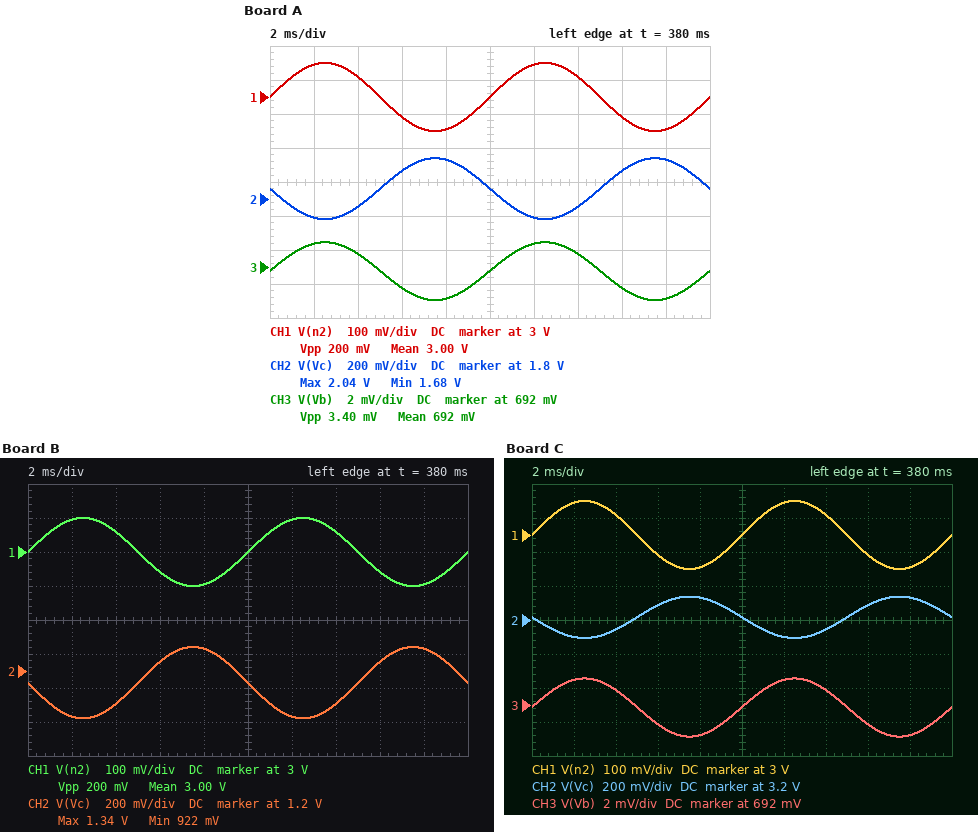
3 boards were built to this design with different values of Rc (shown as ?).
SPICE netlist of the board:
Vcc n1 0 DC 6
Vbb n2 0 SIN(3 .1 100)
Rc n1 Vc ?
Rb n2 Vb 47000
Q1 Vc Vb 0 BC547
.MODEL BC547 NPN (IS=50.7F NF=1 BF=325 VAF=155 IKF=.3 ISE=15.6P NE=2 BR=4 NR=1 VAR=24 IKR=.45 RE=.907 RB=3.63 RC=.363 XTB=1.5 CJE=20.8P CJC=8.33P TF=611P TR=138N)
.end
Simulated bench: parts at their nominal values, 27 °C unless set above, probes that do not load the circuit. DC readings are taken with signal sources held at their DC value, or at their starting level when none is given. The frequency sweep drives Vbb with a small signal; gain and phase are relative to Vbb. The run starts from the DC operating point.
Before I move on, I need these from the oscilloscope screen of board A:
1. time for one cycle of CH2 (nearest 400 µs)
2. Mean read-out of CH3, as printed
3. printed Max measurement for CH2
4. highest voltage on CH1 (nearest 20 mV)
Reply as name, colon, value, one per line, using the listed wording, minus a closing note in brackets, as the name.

time for one cycle of CH2: 10.0 ms
Mean read-out of CH3, as printed: 692 mV
printed Max measurement for CH2: 2.04 V
highest voltage on CH1: 3.10 V
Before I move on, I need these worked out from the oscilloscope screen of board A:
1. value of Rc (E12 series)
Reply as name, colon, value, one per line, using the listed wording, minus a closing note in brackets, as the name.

value of Rc: 330 Ω
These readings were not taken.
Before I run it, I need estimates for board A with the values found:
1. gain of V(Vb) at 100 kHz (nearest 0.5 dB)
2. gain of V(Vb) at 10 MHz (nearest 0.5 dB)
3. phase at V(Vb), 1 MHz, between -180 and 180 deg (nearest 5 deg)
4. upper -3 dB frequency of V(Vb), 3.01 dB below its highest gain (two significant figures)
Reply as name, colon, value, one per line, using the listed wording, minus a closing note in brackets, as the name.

gain of V(Vb) at 100 kHz: -36.0 dB
gain of V(Vb) at 10 MHz: -68.0 dB
phase at V(Vb), 1 MHz, between -180 and 180 deg: -75 deg
upper -3 dB frequency of V(Vb), 3.01 dB below its highest gain: 230 kHz
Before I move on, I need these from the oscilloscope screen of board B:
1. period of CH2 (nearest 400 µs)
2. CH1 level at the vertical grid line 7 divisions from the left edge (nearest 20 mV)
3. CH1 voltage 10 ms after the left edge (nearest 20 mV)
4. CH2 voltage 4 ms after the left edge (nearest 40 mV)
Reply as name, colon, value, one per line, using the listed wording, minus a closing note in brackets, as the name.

period of CH2: 10.0 ms
CH1 level at the vertical grid line 7 divisions from the left edge: 3.06 V
CH1 voltage 10 ms after the left edge: 3.00 V
CH2 voltage 4 ms after the left edge: 1.00 V
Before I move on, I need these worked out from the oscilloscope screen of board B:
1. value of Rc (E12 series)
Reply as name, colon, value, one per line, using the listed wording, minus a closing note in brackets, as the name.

value of Rc: 390 Ω
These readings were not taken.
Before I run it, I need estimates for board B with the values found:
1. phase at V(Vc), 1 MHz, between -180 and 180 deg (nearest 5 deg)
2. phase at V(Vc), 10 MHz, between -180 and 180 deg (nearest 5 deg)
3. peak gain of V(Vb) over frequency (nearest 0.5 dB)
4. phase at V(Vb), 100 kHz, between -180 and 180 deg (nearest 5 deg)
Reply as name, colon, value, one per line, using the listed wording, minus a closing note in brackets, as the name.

phase at V(Vc), 1 MHz, between -180 and 180 deg: 100 deg
phase at V(Vc), 10 MHz, between -180 and 180 deg: 90 deg
peak gain of V(Vb) over frequency: -35.5 dB
phase at V(Vb), 100 kHz, between -180 and 180 deg: -30 deg
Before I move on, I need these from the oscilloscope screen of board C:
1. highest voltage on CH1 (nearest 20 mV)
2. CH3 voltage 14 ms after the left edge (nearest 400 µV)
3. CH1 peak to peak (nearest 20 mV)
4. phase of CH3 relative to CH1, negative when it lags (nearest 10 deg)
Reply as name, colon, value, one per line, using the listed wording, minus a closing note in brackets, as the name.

highest voltage on CH1: 3.10 V
CH3 voltage 14 ms after the left edge: 692.8 mV
CH1 peak to peak: 200 mV
phase of CH3 relative to CH1, negative when it lags: 0 deg
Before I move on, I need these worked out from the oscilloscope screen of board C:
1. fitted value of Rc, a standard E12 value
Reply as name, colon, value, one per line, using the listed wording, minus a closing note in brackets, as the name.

fitted value of Rc, a standard E12 value: 220 Ω
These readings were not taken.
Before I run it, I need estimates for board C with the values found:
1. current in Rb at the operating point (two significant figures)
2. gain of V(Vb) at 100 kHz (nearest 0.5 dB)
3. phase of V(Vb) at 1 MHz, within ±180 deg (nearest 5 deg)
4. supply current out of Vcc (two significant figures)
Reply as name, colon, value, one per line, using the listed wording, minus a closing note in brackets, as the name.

current in Rb at the operating point: 49 µA
gain of V(Vb) at 100 kHz: -35.5 dB
phase of V(Vb) at 1 MHz, within ±180 deg: -70 deg
supply current out of Vcc: 13 mA
